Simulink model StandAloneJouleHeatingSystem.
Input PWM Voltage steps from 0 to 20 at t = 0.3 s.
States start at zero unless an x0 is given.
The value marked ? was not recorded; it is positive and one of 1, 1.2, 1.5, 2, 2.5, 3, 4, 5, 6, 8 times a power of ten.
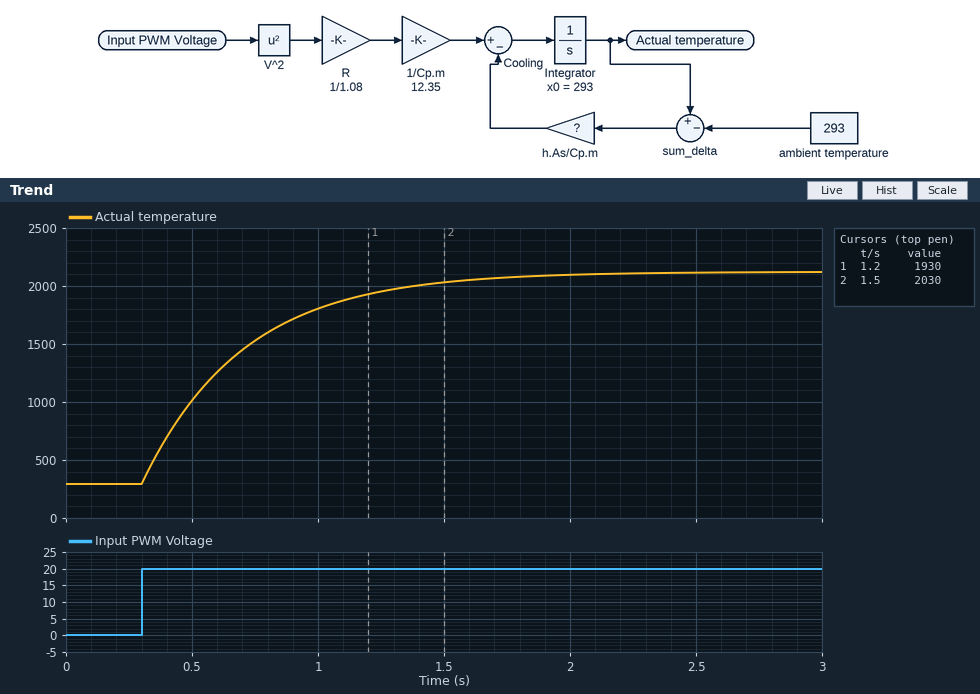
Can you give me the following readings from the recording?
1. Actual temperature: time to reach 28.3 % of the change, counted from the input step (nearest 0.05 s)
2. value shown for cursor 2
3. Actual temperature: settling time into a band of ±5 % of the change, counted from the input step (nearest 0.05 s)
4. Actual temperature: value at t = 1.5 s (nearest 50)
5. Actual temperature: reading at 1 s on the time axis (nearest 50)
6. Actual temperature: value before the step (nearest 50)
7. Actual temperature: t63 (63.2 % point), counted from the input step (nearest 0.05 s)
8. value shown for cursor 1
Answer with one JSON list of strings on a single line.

["0.15 s", "2030", "1.20 s", "2050", "1800", "300", "0.40 s", "1930"]
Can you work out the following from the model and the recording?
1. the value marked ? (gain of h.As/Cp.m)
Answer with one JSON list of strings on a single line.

["2.5"]
